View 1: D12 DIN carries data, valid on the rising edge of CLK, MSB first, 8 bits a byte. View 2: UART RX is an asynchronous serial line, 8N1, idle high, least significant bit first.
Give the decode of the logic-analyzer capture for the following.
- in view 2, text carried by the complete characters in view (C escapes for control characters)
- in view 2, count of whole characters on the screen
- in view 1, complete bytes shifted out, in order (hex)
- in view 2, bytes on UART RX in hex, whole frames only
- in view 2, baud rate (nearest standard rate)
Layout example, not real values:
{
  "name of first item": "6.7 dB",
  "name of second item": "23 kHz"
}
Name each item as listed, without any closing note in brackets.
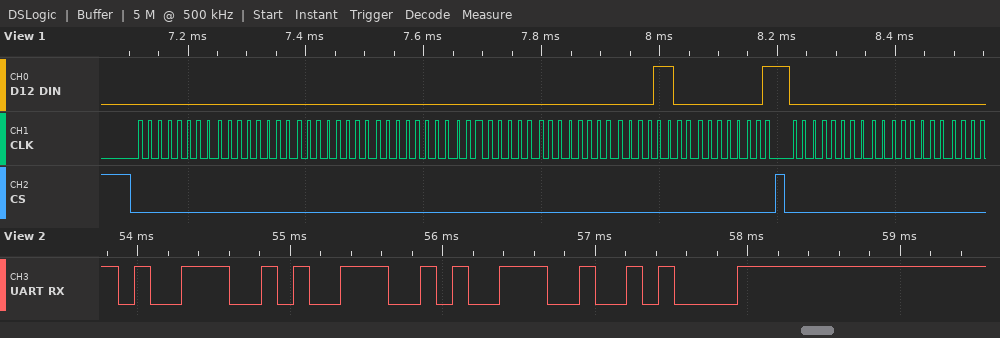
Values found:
{
  "in view 2, text carried by the complete characters in view": "\"999\\n\"",
  "in view 2, count of whole characters on the screen": "4",
  "in view 1, complete bytes shifted out, in order": "00 00 00 00 00 00 0C 01 00 00",
  "in view 2, bytes on UART RX in hex, whole frames only": "39 39 39 0A",
  "in view 2, baud rate": "9600 baud"
}
